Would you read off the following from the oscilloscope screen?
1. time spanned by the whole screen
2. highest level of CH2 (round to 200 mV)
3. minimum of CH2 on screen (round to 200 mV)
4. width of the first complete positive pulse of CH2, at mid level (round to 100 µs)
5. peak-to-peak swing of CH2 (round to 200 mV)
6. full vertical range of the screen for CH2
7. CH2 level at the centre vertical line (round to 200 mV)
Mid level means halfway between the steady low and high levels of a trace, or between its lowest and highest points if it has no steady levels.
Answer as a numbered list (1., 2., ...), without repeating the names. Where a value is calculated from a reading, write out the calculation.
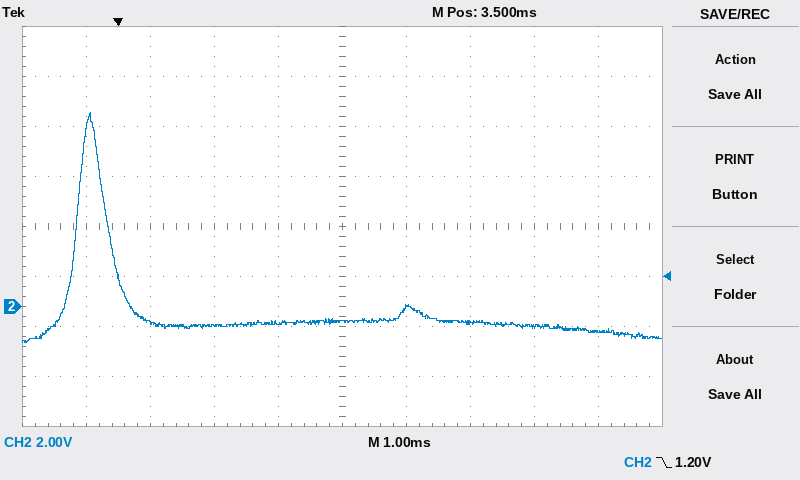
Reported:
1. 10 ms
2. 7.8 V
3. -1.4 V
4. 500 µs
5. 7.8 V − (-1.4 V) = 9.2 V
6. 16 V
7. -600 mV
